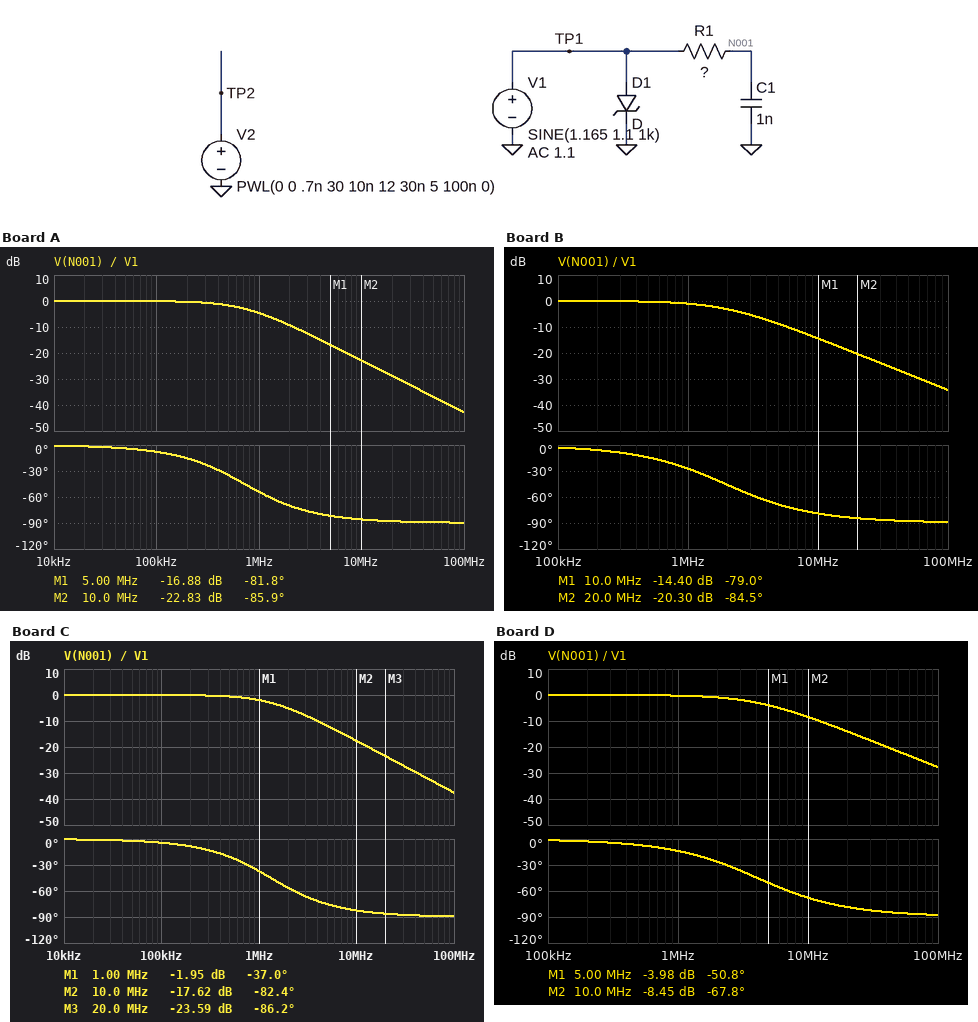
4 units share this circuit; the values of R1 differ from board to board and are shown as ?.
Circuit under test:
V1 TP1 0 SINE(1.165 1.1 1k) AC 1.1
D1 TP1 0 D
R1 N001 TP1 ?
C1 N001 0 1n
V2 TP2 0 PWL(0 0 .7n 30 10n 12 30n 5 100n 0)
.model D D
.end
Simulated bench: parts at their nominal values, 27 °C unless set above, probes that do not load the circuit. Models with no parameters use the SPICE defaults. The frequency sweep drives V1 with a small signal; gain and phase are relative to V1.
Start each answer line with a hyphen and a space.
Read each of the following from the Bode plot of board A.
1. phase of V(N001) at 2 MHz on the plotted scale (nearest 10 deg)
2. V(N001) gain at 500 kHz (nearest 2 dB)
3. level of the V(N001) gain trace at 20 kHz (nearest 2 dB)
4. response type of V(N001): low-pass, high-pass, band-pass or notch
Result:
- -70 deg
- -2 dB
- 0 dB
- low-pass
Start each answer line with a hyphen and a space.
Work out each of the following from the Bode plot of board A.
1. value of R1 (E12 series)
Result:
- 220 Ω
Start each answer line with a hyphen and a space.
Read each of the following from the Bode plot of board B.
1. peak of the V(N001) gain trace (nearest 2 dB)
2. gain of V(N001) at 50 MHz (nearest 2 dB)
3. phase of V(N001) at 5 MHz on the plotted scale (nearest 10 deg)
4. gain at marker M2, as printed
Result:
- 0 dB
- -28 dB
- -70 deg
- -20.30 dB
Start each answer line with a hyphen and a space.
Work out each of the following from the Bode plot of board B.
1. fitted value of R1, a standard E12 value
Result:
- 82 Ω
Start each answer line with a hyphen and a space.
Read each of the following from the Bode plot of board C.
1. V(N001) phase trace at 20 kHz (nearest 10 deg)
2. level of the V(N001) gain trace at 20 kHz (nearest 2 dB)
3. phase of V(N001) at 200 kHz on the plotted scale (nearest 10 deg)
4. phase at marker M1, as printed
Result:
- 0 deg
- 0 dB
- -10 deg
- -37.0 deg
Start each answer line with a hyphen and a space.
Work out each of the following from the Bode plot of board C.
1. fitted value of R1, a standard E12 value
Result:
- 120 Ω
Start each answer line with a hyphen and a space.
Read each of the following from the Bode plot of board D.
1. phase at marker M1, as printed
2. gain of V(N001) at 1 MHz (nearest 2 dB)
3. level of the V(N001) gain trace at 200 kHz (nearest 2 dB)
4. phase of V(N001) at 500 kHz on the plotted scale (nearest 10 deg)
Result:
- -50.8 deg
- 0 dB
- 0 dB
- -10 deg
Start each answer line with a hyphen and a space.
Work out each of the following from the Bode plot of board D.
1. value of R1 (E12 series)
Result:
- 39 Ω
